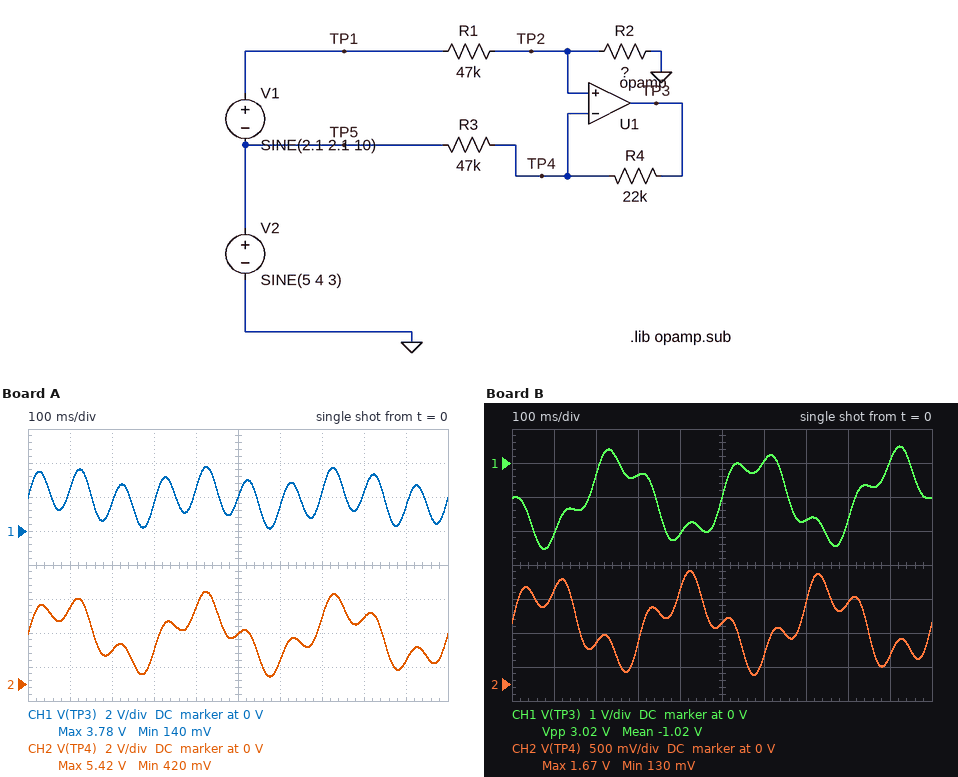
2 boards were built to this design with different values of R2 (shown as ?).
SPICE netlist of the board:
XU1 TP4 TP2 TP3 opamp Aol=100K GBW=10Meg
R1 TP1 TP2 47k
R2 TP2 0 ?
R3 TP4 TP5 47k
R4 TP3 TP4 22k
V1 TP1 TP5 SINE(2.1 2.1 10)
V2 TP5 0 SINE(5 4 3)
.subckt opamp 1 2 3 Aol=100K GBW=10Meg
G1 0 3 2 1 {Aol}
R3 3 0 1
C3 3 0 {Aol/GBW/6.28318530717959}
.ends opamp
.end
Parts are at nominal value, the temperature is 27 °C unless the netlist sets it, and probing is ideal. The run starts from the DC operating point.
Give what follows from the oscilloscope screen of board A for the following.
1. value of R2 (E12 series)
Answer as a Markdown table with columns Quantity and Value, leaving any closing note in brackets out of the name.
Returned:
| Quantity | Value |
|---|---|
| value of R2 | 33 kΩ |
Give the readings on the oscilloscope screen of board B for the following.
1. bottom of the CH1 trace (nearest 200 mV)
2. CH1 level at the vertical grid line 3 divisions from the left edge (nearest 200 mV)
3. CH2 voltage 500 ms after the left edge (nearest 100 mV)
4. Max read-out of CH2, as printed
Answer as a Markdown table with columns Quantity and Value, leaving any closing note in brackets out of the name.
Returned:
| Quantity | Value |
|---|---|
| bottom of the CH1 trace | -2.6 V |
| CH1 level at the vertical grid line 3 divisions from the left edge | -400 mV |
| CH2 voltage 500 ms after the left edge | 900 mV |
| Max read-out of CH2, as printed | 1.67 V |
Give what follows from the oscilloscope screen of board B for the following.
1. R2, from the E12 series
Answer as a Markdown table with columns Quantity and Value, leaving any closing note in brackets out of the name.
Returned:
| Quantity | Value |
|---|---|
| R2, from the E12 series | 6.8 kΩ |
